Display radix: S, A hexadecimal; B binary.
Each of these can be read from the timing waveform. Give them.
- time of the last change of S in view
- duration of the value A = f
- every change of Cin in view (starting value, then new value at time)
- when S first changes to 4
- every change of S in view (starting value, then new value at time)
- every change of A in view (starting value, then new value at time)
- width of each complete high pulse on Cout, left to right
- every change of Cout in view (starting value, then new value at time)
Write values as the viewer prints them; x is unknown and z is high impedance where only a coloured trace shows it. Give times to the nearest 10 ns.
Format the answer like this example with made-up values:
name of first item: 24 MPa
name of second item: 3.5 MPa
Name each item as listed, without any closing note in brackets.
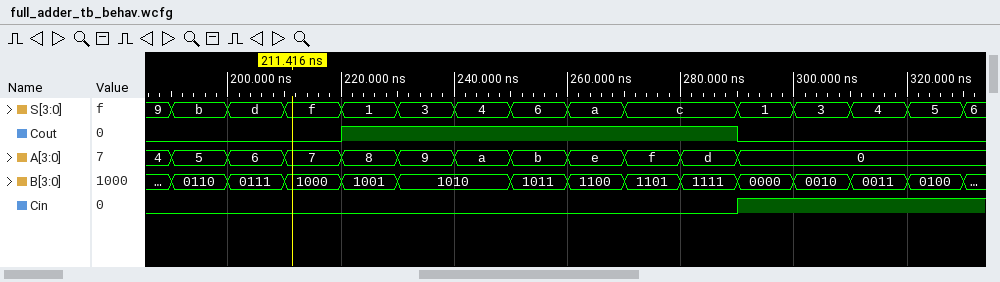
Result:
time of the last change of S in view: 330 ns
duration of the value A = f: 10 ns
every change of Cin in view: 0, 1 at 290 ns
when S first changes to 4: 240 ns
every change of S in view: 9, b at 190 ns, d at 200 ns, f at 210 ns, 1 at 220 ns, 3 at 230 ns, 4 at 240 ns, 6 at 250 ns, a at 260 ns, c at 270 ns, 1 at 290 ns, 3 at 300 ns, 4 at 310 ns, 5 at 320 ns, 6 at 330 ns
every change of A in view: 4, 5 at 190 ns, 6 at 200 ns, 7 at 210 ns, 8 at 220 ns, 9 at 230 ns, a at 240 ns, b at 250 ns, e at 260 ns, f at 270 ns, d at 280 ns, 0 at 290 ns
width of each complete high pulse on Cout, left to right: 70 ns
every change of Cout in view: 0, 1 at 220 ns, 0 at 290 ns
